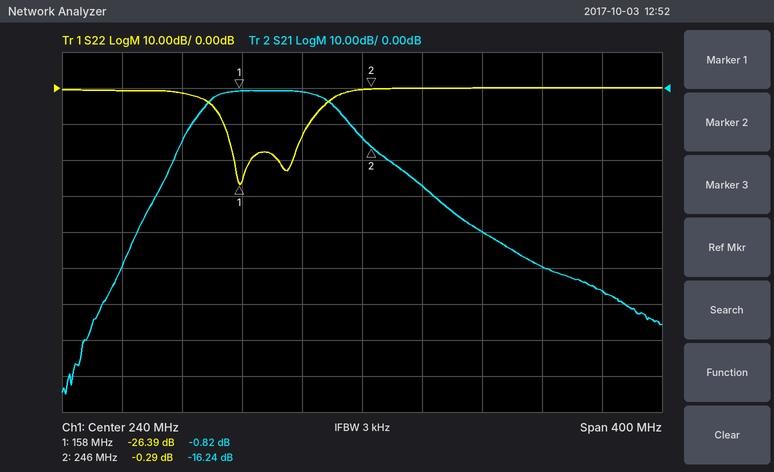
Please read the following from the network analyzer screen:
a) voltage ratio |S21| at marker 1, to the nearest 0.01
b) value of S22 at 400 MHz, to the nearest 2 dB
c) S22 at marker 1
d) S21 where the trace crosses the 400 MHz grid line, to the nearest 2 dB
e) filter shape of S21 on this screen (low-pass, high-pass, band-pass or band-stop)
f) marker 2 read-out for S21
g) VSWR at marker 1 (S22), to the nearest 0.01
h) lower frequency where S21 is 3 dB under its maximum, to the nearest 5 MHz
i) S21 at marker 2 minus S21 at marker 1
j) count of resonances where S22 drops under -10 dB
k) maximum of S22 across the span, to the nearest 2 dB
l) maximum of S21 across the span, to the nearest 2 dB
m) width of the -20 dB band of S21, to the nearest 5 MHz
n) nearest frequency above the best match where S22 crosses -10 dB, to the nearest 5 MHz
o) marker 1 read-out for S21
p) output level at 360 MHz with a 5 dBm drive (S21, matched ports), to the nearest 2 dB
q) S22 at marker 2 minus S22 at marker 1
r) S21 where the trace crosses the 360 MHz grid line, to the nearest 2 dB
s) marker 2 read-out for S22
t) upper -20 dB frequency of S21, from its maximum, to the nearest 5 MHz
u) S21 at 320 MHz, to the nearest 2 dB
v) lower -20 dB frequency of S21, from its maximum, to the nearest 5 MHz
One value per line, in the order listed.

0.91
0 dB
-26.39 dB
-56 dB
band-pass
-16.24 dB
1.10
140 MHz
-15.42 dB
2
0 dB
0 dB
145 MHz
205 MHz
-0.82 dB
-44 dBm
26.10 dB
-50 dB
-0.29 dB
260 MHz
-40 dB
115 MHz
